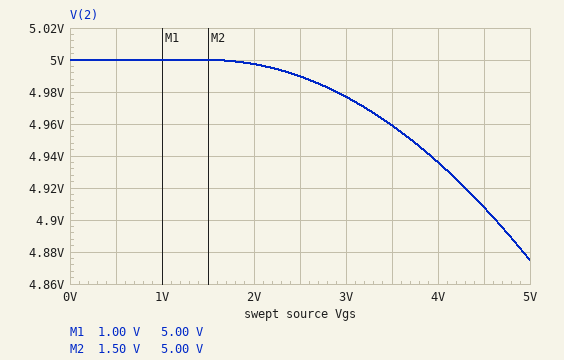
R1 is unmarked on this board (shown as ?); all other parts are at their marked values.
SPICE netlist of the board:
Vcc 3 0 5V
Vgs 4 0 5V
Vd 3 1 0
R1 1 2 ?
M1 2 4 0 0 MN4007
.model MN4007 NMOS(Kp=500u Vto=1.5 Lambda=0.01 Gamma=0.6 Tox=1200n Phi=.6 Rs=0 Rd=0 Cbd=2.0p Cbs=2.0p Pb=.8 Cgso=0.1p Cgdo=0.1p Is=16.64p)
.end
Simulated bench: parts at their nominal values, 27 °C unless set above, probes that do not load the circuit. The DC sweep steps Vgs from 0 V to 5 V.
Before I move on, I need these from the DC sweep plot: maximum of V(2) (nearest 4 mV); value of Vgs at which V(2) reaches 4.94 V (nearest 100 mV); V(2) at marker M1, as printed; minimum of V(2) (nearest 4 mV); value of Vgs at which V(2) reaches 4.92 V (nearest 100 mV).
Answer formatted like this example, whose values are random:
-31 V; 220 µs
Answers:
5.000 V; 3.9 V; 5.00 V; 4.876 V; 4.3 V
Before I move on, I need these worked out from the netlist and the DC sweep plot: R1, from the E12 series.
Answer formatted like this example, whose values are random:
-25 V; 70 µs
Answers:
39 Ω
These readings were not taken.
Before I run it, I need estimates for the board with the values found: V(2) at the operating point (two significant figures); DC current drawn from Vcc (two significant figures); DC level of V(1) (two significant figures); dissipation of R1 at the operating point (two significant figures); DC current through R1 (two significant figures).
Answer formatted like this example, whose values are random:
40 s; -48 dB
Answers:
4.9 V; 3.2 mA; 5.0 V; 400 µW; 3.2 mA
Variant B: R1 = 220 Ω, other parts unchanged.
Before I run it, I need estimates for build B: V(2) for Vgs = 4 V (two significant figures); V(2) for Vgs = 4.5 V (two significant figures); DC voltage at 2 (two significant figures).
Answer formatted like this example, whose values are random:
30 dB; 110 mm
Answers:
4.6 V; 4.5 V; 4.3 V
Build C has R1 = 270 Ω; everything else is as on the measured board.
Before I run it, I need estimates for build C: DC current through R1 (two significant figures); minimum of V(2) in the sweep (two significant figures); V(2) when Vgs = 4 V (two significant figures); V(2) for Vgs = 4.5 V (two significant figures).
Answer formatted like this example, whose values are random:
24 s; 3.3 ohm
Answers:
3.2 mA; 4.1 V; 4.6 V; 4.4 V
